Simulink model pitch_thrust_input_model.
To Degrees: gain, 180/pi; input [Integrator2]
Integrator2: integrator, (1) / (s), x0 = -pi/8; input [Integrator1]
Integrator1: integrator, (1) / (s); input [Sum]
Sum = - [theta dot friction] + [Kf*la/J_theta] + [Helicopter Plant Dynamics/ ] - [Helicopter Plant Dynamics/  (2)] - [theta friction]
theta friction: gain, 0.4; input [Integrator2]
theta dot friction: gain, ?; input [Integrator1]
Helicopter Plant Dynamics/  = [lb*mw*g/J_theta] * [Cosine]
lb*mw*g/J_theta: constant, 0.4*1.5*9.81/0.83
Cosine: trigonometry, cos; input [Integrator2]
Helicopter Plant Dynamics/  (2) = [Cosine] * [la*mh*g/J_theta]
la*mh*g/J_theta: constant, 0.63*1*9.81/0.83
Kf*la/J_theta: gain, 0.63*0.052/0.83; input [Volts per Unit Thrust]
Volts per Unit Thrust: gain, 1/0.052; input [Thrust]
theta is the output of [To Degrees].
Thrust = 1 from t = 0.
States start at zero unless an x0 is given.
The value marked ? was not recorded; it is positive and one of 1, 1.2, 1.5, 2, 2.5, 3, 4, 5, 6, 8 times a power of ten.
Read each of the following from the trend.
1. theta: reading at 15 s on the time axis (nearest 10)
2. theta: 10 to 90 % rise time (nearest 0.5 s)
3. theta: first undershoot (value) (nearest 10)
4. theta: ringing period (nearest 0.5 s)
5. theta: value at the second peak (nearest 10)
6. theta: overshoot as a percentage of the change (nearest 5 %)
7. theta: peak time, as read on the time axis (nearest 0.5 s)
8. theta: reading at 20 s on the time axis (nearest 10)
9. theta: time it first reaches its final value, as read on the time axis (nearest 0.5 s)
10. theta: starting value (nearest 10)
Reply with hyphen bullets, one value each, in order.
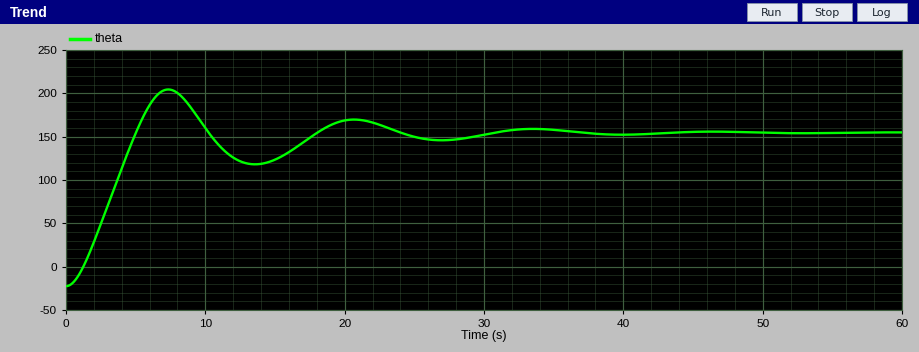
- 120
- 3.5 s
- 120
- 13.5 s
- 170
- 30 %
- 7.5 s
- 170
- 5.0 s
- -20
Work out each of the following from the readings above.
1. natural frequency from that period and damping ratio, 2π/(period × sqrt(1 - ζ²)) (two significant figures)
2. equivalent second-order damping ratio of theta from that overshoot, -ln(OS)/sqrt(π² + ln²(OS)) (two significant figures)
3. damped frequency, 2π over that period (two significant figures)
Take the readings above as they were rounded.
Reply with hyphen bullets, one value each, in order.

- 0.50 rad/s
- 0.36
- 0.47 rad/s
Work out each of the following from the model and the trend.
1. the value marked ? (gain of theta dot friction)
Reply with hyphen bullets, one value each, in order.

- 0.2
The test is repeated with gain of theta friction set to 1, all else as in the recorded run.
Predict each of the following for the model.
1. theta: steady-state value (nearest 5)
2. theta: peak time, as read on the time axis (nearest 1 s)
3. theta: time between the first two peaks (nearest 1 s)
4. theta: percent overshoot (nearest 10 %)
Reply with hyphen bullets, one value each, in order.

- 25
- 3 s
- 7 s
- 80 %
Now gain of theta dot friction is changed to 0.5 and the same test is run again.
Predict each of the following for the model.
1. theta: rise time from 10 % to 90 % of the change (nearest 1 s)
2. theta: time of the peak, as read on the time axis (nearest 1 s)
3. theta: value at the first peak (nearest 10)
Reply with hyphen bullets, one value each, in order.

- 6 s
- 11 s
- 160
